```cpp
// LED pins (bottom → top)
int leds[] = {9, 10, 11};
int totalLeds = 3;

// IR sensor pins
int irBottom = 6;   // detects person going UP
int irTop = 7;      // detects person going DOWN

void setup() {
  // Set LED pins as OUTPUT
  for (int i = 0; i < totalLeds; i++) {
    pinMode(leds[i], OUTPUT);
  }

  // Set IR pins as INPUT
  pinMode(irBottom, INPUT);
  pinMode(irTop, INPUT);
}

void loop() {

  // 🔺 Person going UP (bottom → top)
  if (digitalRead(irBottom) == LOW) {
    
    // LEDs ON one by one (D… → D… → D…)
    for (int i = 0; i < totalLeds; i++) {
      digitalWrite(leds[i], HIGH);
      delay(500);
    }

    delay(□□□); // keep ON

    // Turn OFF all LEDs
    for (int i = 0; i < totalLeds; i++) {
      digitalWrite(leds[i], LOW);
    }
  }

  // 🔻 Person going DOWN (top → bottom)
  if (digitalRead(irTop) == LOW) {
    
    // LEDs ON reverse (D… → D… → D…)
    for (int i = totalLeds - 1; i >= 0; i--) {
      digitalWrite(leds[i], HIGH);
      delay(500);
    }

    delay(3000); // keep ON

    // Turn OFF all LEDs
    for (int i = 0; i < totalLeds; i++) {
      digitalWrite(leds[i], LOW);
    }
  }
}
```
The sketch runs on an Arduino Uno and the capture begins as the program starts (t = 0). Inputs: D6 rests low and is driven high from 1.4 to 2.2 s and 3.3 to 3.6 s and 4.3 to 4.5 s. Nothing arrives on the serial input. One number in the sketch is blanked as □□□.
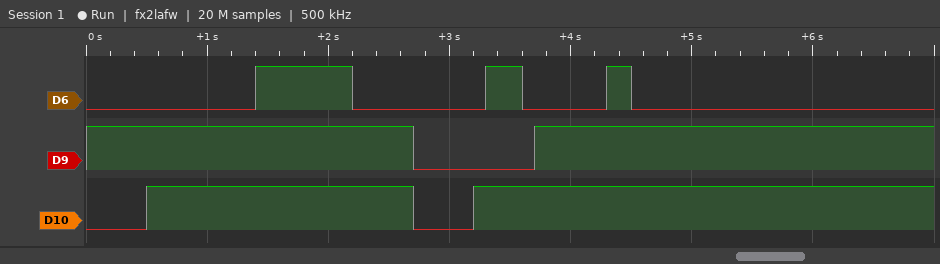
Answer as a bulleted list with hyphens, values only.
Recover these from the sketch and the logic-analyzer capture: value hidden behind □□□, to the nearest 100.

- 1200
